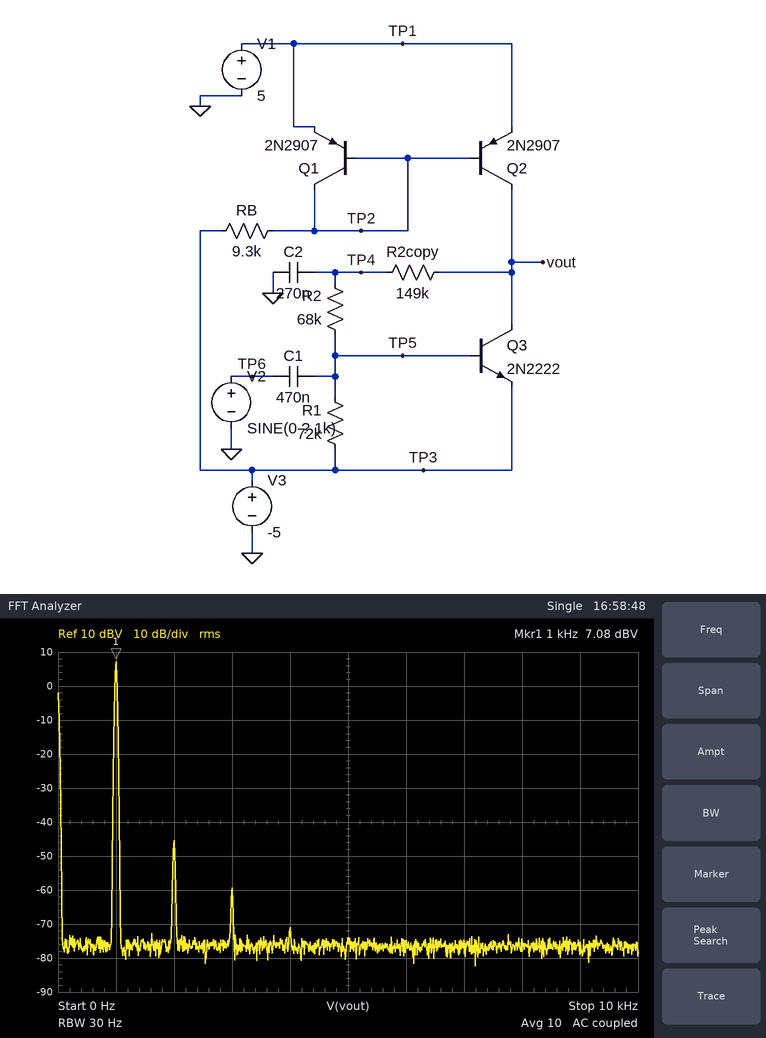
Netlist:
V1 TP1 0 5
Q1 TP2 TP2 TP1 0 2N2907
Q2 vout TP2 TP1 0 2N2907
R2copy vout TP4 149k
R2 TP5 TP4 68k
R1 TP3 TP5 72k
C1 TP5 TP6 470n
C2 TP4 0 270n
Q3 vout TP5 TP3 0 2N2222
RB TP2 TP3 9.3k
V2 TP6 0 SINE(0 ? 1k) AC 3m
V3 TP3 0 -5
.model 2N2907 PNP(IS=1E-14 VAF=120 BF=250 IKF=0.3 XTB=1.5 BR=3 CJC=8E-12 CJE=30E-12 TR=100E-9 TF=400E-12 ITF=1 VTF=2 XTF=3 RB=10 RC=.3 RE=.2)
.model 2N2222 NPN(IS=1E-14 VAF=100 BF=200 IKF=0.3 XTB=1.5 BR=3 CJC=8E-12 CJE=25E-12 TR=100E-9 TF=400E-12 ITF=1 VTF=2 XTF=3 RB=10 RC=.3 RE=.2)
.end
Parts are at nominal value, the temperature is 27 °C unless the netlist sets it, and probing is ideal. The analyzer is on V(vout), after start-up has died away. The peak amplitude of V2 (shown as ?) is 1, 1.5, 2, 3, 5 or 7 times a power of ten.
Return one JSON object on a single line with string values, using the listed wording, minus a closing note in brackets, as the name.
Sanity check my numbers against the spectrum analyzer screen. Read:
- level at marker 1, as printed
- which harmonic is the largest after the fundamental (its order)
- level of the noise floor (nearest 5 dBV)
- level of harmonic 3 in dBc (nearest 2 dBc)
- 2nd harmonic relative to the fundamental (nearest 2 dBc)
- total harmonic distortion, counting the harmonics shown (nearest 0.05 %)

{"level at marker 1, as printed": "7.08 dBV", "which harmonic is the largest after the fundamental": "2", "level of the noise floor": "-75 dBV", "level of harmonic 3 in dBc": "-66 dBc", "2nd harmonic relative to the fundamental": "-52 dBc", "total harmonic distortion, counting the harmonics shown": "0.25 %"}
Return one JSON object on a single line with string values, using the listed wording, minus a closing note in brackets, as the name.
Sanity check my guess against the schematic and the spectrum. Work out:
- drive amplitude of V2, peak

{"drive amplitude of V2, peak": "2 mV"}
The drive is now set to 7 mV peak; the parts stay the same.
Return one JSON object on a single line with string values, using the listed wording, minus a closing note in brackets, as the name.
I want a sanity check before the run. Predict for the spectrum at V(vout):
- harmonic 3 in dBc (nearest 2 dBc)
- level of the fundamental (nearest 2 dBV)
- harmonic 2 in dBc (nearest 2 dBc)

{"harmonic 3 in dBc": "-14 dBc", "level of the fundamental": "12 dBV", "harmonic 2 in dBc": "-20 dBc"}
